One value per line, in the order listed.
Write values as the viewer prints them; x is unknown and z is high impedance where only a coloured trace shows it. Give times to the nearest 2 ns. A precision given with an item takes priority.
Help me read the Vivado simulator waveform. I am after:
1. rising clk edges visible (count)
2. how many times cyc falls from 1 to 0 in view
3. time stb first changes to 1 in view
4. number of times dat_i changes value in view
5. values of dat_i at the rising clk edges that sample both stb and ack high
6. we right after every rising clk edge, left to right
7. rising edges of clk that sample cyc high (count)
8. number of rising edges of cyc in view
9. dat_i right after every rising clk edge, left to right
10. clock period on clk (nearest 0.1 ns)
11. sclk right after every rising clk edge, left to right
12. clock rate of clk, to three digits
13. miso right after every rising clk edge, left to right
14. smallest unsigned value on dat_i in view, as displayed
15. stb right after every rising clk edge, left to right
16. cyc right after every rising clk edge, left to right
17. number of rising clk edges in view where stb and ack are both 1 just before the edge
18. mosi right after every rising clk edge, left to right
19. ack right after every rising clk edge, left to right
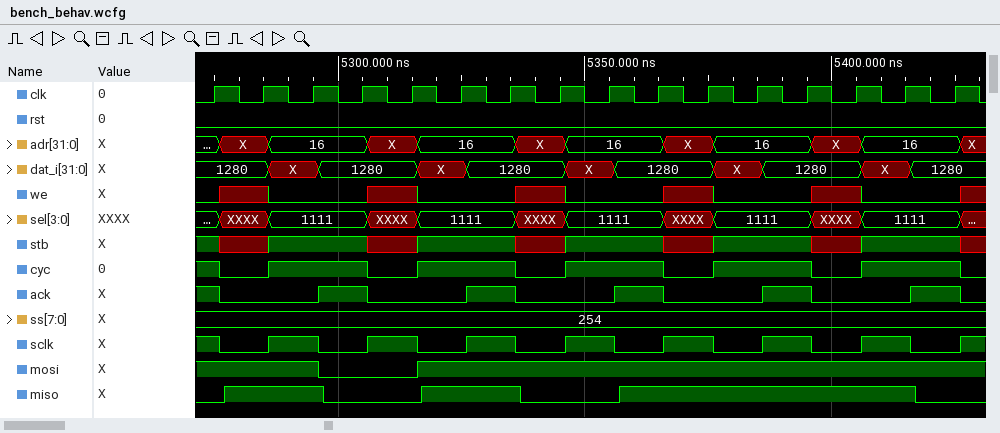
16
6
5286 ns
10
1280, 1280, 1280, 1280, 1280, 1280
0 x 0 0 x 0 0 x 0 0 x 0 0 x 0 0
11
5
1280, 1280, X, 1280, 1280, X, 1280, 1280, X, 1280, 1280, X, 1280, 1280, X, 1280
10 ns
1 0 1 0 1 0 1 0 1 0 1 0 1 0 1 0
100 MHz
0 1 1 0 0 1 1 0 0 1 1 1 1 1 1 0
1280
1 x 1 1 x 1 1 x 1 1 x 1 1 x 1 1
1 0 1 1 0 1 1 0 1 1 0 1 1 0 1 1
6
1 1 1 0 0 1 1 1 1 1 1 1 1 1 1 1
1 0 0 1 0 0 1 0 0 1 0 0 1 0 0 1
